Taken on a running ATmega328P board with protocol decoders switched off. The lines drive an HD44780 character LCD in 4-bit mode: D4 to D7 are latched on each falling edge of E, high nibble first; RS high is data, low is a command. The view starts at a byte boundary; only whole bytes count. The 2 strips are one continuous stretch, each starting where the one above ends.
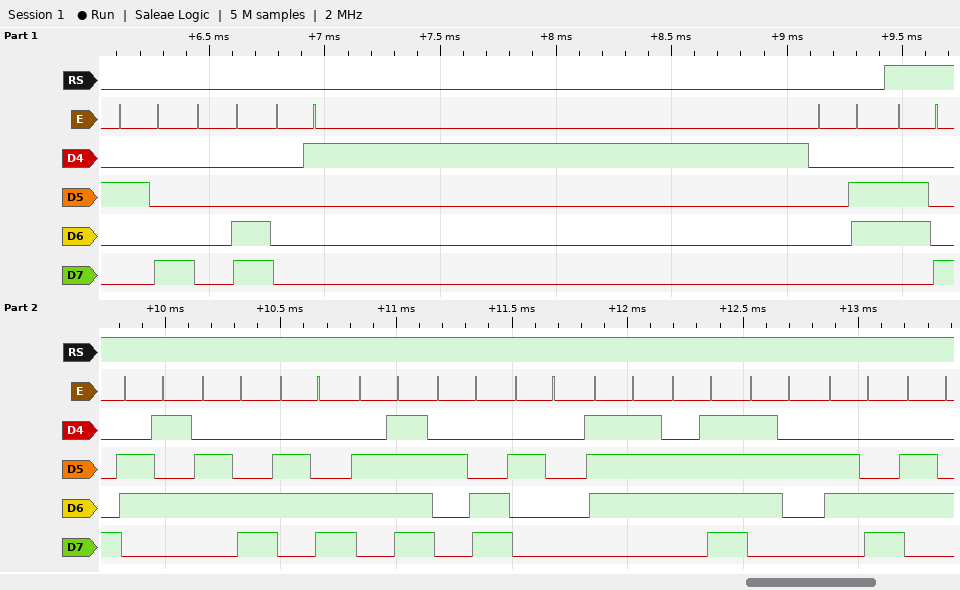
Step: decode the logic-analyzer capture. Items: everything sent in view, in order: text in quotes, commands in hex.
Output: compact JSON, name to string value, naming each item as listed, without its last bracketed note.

{"everything sent in view, in order: text in quotes, commands in hex": "0x28 0x0C 0x01 0x06 \"hello, world\""}
